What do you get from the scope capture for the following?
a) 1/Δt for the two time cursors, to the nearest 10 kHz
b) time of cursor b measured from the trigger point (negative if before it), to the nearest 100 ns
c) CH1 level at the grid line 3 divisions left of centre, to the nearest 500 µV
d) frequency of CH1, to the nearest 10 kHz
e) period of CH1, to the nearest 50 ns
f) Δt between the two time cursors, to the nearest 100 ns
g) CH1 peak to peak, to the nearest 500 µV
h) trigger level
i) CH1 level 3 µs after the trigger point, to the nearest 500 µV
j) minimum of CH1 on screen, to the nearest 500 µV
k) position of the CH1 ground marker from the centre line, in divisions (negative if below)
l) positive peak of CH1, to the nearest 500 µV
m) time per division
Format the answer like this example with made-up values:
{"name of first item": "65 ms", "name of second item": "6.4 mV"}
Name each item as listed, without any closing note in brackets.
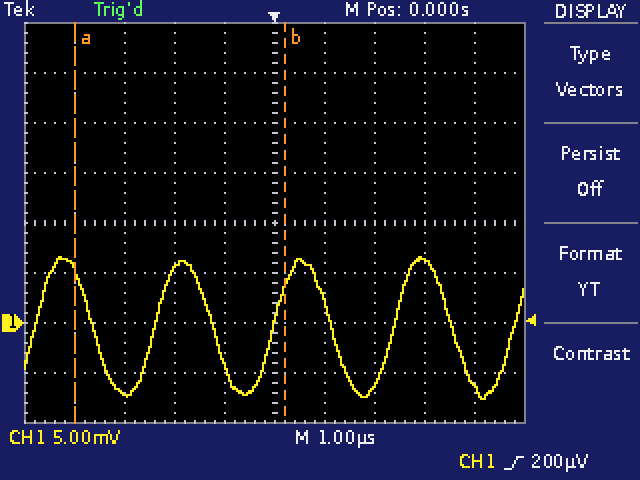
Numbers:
{"1/Δt for the two time cursors, to the nearest 10 kHz": "240 kHz", "time of cursor b measured from the trigger point (negative if before it), to the nearest 100 ns": "+200 ns", "CH1 level at the grid line 3 divisions left of centre, to the nearest 500 µV": "-7.0 mV", "frequency of CH1, to the nearest 10 kHz": "420 kHz", "period of CH1, to the nearest 50 ns": "2.40 µs", "Δt between the two time cursors, to the nearest 100 ns": "4.2 µs", "CH1 peak to peak, to the nearest 500 µV": "14.0 mV", "trigger level": "200 µV", "CH1 level 3 µs after the trigger point, to the nearest 500 µV": "6.5 mV", "minimum of CH1 on screen, to the nearest 500 µV": "-7.5 mV", "position of the CH1 ground marker from the centre line, in divisions": "-2.0 div", "positive peak of CH1, to the nearest 500 µV": "6.5 mV", "time per division": "1 µs"}
